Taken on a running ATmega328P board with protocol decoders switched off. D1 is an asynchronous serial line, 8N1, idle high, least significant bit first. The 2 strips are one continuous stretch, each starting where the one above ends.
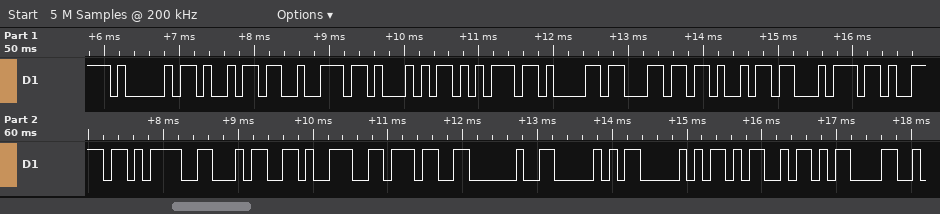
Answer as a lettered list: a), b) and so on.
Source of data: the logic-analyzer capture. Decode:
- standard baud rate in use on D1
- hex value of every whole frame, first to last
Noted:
a) 9600 baud
b) 41 69 72 51 75 61 6C 69 74 79 3D 34 39 37 20 50 50 4D 0D
